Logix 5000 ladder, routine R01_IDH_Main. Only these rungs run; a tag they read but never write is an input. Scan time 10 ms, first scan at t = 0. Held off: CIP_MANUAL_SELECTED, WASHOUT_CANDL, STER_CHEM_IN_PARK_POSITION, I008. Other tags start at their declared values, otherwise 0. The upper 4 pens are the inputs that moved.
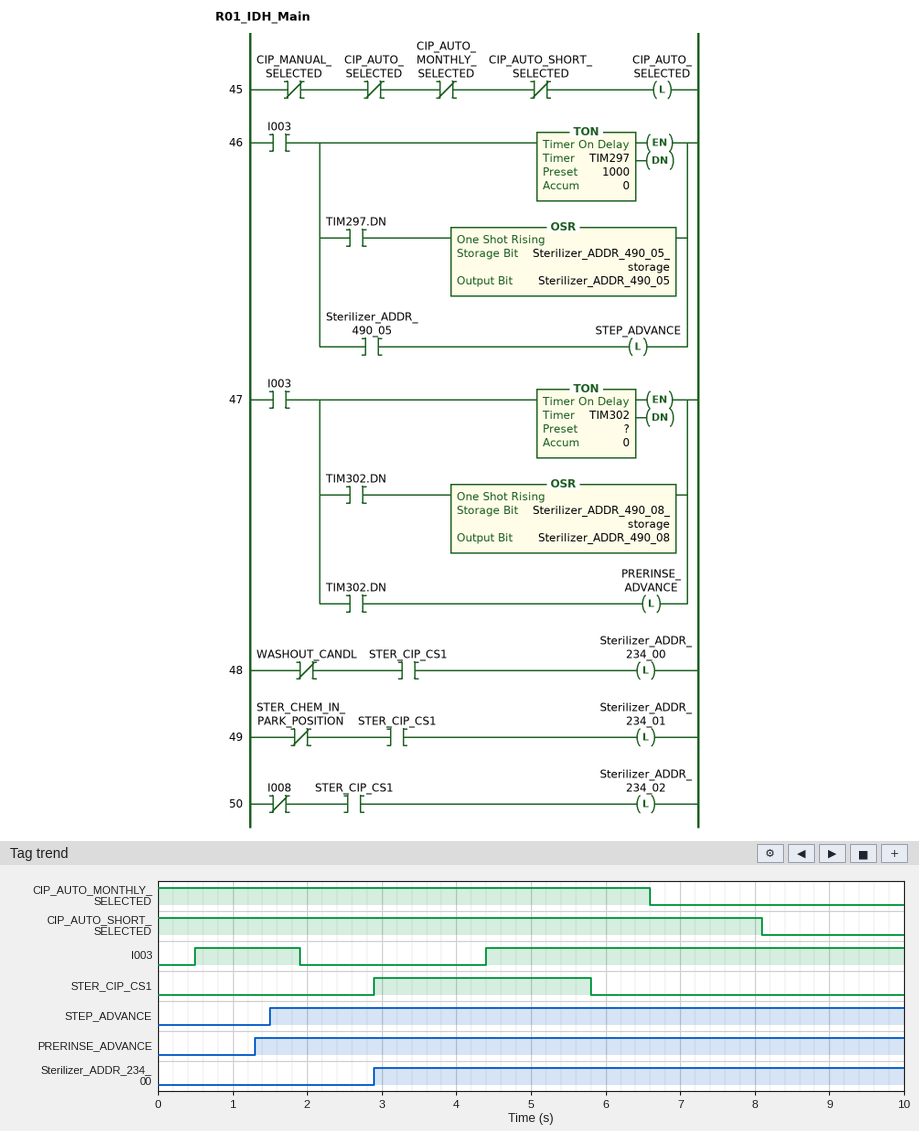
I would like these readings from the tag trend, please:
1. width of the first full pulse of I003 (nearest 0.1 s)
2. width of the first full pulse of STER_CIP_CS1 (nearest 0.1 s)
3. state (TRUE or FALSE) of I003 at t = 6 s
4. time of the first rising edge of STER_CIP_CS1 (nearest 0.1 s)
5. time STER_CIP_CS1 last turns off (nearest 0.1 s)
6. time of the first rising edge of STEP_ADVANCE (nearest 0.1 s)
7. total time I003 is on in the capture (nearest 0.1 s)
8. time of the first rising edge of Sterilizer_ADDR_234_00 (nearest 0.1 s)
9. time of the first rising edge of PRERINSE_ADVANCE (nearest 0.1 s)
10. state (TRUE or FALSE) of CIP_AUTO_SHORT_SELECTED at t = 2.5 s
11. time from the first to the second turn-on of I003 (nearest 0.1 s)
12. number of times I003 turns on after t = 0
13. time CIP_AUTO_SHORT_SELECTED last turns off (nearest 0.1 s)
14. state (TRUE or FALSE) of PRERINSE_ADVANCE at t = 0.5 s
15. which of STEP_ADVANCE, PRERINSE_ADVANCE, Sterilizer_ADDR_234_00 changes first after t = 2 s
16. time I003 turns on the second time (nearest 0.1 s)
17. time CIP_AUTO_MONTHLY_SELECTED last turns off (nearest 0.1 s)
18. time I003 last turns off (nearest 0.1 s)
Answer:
1.4 s
2.9 s
TRUE
2.9 s
5.8 s
1.5 s
7.0 s
2.9 s
1.3 s
TRUE
3.9 s
2
8.1 s
FALSE
Sterilizer_ADDR_234_00
4.4 s
6.6 s
1.9 s
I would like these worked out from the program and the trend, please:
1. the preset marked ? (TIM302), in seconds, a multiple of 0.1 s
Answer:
0.8 s
